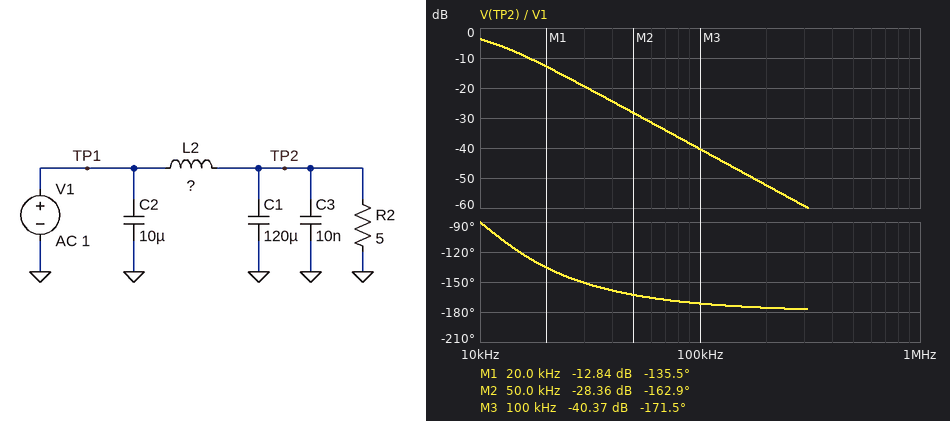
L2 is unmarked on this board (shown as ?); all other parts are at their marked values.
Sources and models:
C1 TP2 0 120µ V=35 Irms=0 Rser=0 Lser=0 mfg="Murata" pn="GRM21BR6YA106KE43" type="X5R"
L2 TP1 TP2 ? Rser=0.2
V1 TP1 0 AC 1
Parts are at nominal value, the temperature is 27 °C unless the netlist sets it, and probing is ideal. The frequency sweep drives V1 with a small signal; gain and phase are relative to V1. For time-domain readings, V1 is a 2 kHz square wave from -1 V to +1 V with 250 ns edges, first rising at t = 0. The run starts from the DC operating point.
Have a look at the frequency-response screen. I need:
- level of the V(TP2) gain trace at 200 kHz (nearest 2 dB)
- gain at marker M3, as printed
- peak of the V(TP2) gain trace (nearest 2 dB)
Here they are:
-52 dB
-40.37 dB
-4 dB
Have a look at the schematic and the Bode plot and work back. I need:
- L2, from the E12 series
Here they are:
2.2 µH
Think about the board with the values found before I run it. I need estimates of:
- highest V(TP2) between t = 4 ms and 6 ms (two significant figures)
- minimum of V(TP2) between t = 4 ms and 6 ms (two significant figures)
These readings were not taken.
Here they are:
1.0 V
-1.0 V
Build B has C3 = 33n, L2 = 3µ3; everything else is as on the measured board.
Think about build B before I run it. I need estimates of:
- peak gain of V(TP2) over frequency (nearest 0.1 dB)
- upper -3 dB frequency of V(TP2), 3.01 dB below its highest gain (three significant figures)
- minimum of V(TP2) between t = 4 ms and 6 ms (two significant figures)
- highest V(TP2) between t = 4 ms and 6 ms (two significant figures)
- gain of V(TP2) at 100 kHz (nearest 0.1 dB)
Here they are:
0 dB
9.03 kHz
-1.1 V
1.1 V
-43.9 dB
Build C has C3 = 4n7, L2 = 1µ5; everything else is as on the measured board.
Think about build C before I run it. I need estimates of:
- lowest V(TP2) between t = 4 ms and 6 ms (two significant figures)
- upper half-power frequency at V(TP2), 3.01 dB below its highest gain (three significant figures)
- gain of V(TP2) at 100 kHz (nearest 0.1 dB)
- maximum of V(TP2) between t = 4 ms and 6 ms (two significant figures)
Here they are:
-970 mV
9.19 kHz
-37.1 dB
970 mV
